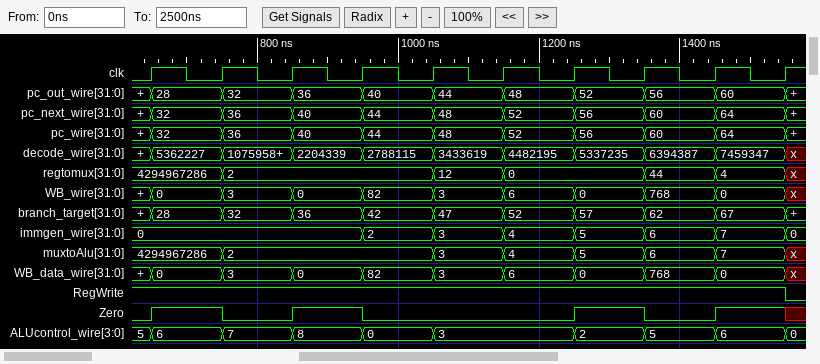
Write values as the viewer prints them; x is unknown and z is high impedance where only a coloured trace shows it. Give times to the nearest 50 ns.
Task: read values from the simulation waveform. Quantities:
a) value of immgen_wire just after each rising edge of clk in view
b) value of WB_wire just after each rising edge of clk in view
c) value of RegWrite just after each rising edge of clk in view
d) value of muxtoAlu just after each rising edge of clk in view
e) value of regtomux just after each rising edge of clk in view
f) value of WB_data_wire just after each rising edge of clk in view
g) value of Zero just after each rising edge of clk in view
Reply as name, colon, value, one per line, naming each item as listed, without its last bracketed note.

value of immgen_wire just after each rising edge of clk in view: 0, 0, 0, 2, 3, 4, 5, 6, 7, 0
value of WB_wire just after each rising edge of clk in view: 0, 3, 0, 82, 3, 6, 0, 768, 0, x
value of RegWrite just after each rising edge of clk in view: 1 1 1 1 1 1 1 1 1 0
value of muxtoAlu just after each rising edge of clk in view: 4294967286, 2, 2, 2, 3, 4, 5, 6, 7, x
value of regtomux just after each rising edge of clk in view: 4294967286, 2, 2, 2, 12, 0, 0, 44, 4, x
value of WB_data_wire just after each rising edge of clk in view: 0, 3, 0, 82, 3, 6, 0, 768, 0, x
value of Zero just after each rising edge of clk in view: 1 0 1 0 0 0 1 0 1 x
